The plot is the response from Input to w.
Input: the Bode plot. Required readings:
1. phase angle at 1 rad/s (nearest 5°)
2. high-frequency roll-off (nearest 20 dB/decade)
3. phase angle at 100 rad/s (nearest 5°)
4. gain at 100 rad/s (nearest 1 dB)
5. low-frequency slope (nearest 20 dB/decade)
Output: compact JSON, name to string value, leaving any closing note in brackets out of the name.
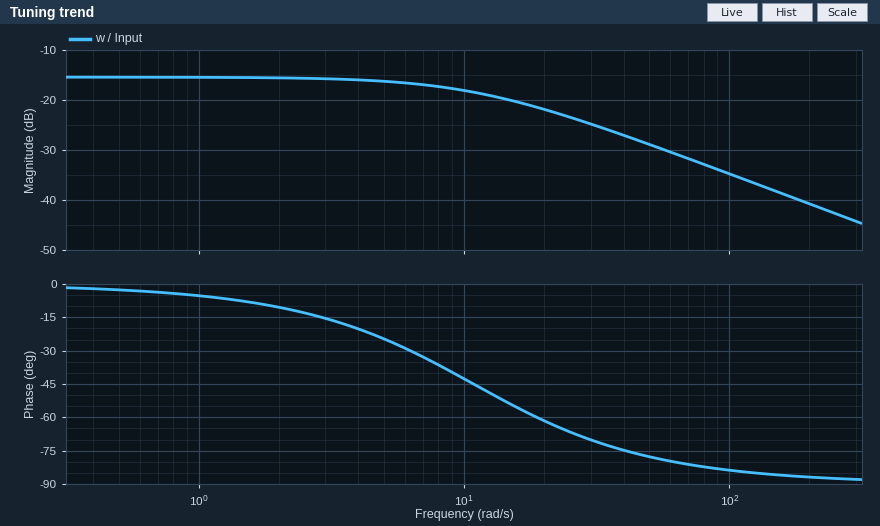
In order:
{"phase angle at 1 rad/s": "-5°", "high-frequency roll-off": "-20 dB/decade", "phase angle at 100 rad/s": "-85°", "gain at 100 rad/s": "-35 dB", "low-frequency slope": "0 dB/decade"}
